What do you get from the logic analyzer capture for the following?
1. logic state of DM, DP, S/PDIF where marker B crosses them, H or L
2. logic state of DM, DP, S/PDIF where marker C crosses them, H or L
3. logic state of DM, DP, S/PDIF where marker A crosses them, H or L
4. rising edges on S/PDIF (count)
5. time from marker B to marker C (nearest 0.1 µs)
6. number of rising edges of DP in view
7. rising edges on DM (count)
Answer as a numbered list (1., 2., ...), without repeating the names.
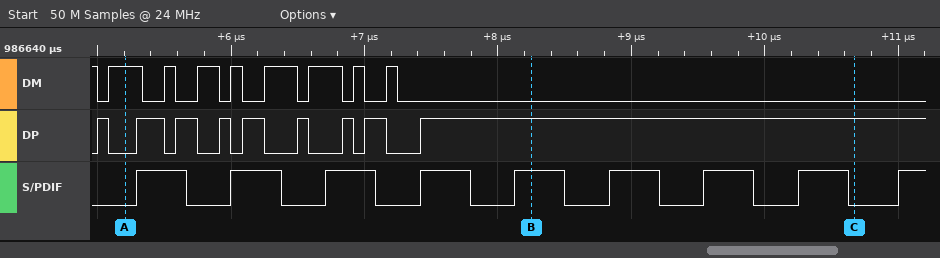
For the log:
1. DM=L, DP=H, S/PDIF=H
2. DM=L, DP=H, S/PDIF=L
3. DM=H, DP=L, S/PDIF=L
4. 9
5. 2.4 µs
6. 9
7. 8
